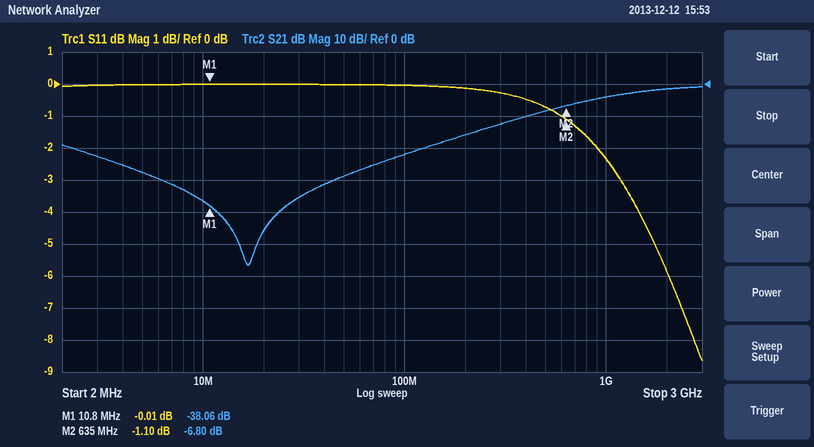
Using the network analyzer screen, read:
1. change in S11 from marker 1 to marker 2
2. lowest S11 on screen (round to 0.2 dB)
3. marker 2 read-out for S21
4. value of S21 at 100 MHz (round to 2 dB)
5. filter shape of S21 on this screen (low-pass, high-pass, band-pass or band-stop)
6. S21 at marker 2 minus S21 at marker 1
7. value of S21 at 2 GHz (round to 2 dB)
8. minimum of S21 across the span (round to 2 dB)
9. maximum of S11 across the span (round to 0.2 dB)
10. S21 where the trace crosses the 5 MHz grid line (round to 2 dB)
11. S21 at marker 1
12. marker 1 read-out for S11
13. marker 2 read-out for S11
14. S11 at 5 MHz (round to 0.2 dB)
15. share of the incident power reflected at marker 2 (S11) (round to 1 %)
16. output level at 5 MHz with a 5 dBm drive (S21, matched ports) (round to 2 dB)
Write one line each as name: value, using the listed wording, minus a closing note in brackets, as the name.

change in S11 from marker 1 to marker 2: -1.09 dB
lowest S11 on screen: -8.6 dB
marker 2 read-out for S21: -6.80 dB
value of S21 at 100 MHz: -22 dB
filter shape of S21 on this screen: high-pass
S21 at marker 2 minus S21 at marker 1: 31.26 dB
value of S21 at 2 GHz: -2 dB
minimum of S21 across the span: -56 dB
maximum of S11 across the span: 0.0 dB
S21 where the trace crosses the 5 MHz grid line: -28 dB
S21 at marker 1: -38.06 dB
marker 1 read-out for S11: -0.01 dB
marker 2 read-out for S11: -1.10 dB
S11 at 5 MHz: 0.0 dB
share of the incident power reflected at marker 2 (S11): 78 %
output level at 5 MHz with a 5 dBm drive (S21, matched ports): -22 dBm
